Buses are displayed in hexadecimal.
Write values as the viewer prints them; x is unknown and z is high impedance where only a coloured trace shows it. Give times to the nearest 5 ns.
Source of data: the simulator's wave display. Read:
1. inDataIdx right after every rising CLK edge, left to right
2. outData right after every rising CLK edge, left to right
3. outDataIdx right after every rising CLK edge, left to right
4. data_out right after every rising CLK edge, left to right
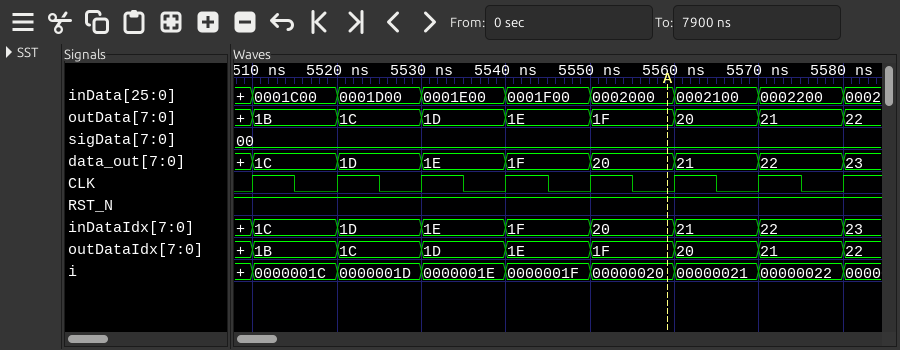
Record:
1C, 1D, 1E, 1F, 20, 21, 22, 23
1B, 1C, 1D, 1E, 1F, 20, 21, 22
1B, 1C, 1D, 1E, 1F, 20, 21, 22
1C, 1D, 1E, 1F, 20, 21, 22, 23
